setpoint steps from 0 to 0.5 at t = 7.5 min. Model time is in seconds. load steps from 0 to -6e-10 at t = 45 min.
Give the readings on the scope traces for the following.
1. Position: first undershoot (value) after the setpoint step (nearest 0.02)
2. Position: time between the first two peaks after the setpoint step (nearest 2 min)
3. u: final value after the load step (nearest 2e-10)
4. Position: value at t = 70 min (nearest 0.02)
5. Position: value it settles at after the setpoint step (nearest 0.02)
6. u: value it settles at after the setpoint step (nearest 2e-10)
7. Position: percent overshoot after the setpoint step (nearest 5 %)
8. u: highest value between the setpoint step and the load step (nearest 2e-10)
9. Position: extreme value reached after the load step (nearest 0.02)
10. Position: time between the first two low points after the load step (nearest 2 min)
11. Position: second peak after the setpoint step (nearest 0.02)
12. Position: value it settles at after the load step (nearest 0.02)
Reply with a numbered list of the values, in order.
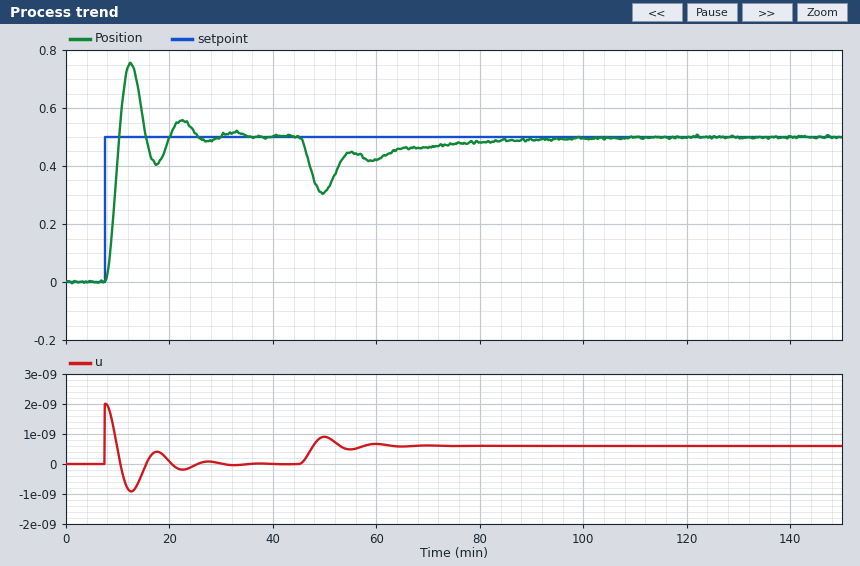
1. 0.40
2. 10 min
3. 0.0000000006
4. 0.46
5. 0.50
6. 0.0000000000
7. 50 %
8. 0.0000000020
9. 0.30
10. 10 min
11. 0.56
12. 0.50
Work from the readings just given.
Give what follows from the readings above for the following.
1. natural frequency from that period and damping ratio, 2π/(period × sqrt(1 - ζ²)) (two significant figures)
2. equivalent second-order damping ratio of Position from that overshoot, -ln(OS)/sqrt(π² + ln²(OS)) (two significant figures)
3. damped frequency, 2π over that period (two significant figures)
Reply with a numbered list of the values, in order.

1. 0.64 rad/min
2. 0.22
3. 0.63 rad/min
